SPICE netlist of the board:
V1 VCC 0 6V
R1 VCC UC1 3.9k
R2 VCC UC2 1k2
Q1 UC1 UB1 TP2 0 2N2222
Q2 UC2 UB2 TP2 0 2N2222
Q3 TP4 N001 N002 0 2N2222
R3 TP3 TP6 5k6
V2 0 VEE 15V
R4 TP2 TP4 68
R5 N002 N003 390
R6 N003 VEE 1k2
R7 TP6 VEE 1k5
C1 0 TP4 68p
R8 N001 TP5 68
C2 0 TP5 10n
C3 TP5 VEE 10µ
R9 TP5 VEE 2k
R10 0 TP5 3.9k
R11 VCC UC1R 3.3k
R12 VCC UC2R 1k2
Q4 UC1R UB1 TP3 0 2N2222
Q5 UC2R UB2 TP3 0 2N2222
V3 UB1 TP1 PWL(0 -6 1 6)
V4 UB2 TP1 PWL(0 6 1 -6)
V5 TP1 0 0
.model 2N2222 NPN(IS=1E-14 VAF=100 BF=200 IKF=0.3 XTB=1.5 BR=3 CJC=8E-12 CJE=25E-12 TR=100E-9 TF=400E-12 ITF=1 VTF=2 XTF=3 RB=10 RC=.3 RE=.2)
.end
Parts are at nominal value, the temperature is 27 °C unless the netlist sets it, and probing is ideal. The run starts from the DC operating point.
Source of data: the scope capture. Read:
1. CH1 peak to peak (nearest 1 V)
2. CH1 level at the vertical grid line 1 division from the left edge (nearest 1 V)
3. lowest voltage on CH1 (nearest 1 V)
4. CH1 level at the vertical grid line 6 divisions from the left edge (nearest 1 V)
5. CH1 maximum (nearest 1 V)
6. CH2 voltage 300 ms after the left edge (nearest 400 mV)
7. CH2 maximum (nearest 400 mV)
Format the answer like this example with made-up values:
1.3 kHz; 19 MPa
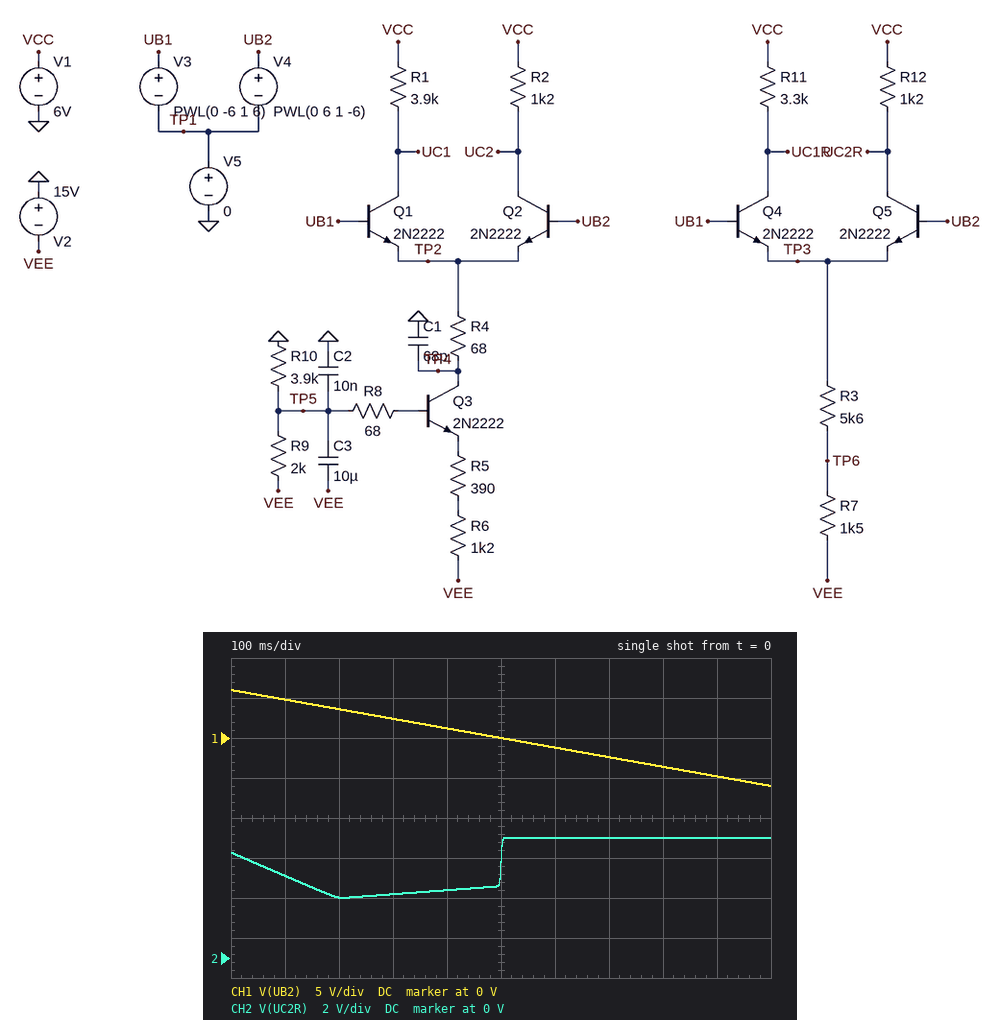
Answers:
12 V; 5 V; -6 V; -1 V; 6 V; 3.2 V; 6.0 V
